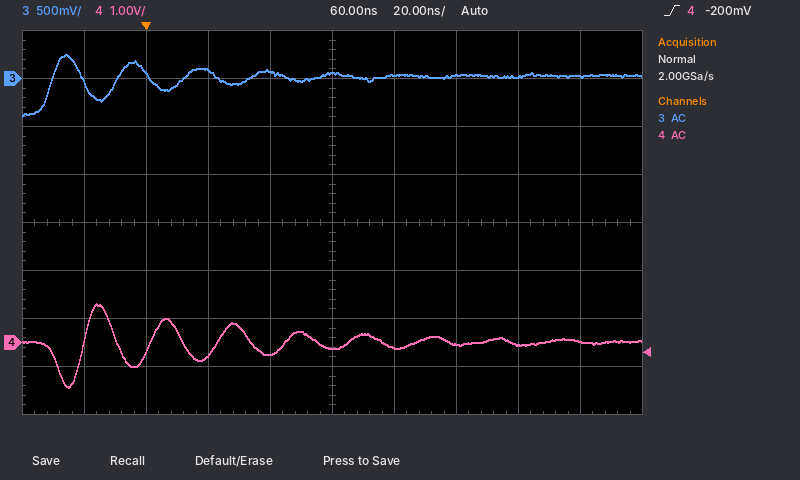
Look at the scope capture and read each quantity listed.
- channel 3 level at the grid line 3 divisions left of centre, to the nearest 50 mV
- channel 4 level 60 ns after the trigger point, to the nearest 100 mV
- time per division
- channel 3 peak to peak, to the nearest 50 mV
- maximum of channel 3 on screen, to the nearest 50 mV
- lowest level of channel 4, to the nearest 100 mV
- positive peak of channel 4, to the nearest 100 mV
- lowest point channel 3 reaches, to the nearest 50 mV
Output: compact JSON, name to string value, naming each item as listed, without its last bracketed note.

{"channel 3 level at the grid line 3 divisions left of centre, to the nearest 50 mV": "50 mV", "channel 4 level 60 ns after the trigger point, to the nearest 100 mV": "-100 mV", "time per division": "20 ns", "channel 3 peak to peak, to the nearest 50 mV": "650 mV", "maximum of channel 3 on screen, to the nearest 50 mV": "250 mV", "lowest level of channel 4, to the nearest 100 mV": "-900 mV", "positive peak of channel 4, to the nearest 100 mV": "800 mV", "lowest point channel 3 reaches, to the nearest 50 mV": "-400 mV"}
